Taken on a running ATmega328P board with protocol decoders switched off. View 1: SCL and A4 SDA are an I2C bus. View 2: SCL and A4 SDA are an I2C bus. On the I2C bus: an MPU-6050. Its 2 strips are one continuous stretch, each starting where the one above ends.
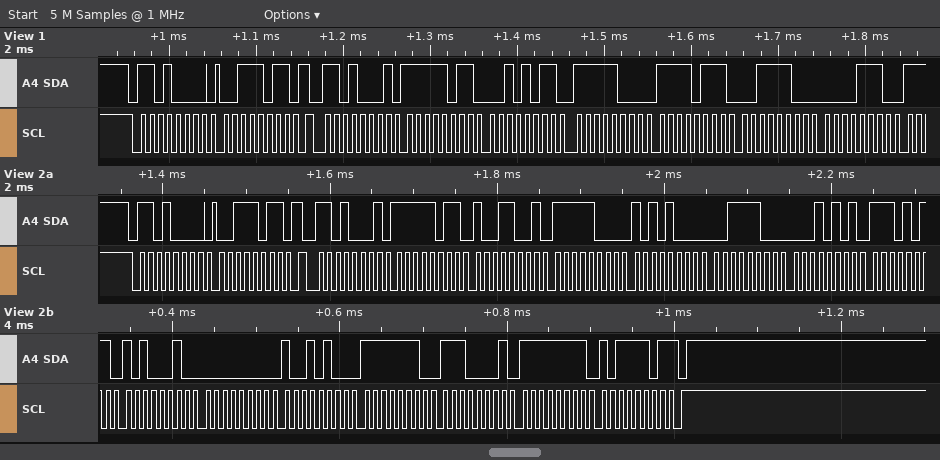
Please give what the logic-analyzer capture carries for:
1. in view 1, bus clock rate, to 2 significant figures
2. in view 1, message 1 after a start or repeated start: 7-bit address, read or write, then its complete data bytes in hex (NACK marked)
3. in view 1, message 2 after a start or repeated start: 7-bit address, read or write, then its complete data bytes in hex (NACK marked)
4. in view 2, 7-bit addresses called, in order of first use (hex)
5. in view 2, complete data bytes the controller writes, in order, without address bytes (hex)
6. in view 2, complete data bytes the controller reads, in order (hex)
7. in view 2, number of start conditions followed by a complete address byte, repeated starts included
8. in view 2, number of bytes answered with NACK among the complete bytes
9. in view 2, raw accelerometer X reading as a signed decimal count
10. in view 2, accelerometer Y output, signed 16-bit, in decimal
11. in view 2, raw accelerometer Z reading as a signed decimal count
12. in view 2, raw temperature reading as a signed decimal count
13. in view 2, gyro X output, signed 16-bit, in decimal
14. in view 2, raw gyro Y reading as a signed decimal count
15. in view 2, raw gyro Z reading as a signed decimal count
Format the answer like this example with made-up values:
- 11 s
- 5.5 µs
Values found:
- 100 kHz
- 0x68 write: 3B
- 0x68 read: FB 2B F8 F7 3C 0E
- 0x68
- 3B
- FB 99 F8 A8 3C 15 EB A2 00 94 FE E1 FF BD
- 2
- 1
- -1127
- -1880
- 15381
- -5214
- 148
- -287
- -67
